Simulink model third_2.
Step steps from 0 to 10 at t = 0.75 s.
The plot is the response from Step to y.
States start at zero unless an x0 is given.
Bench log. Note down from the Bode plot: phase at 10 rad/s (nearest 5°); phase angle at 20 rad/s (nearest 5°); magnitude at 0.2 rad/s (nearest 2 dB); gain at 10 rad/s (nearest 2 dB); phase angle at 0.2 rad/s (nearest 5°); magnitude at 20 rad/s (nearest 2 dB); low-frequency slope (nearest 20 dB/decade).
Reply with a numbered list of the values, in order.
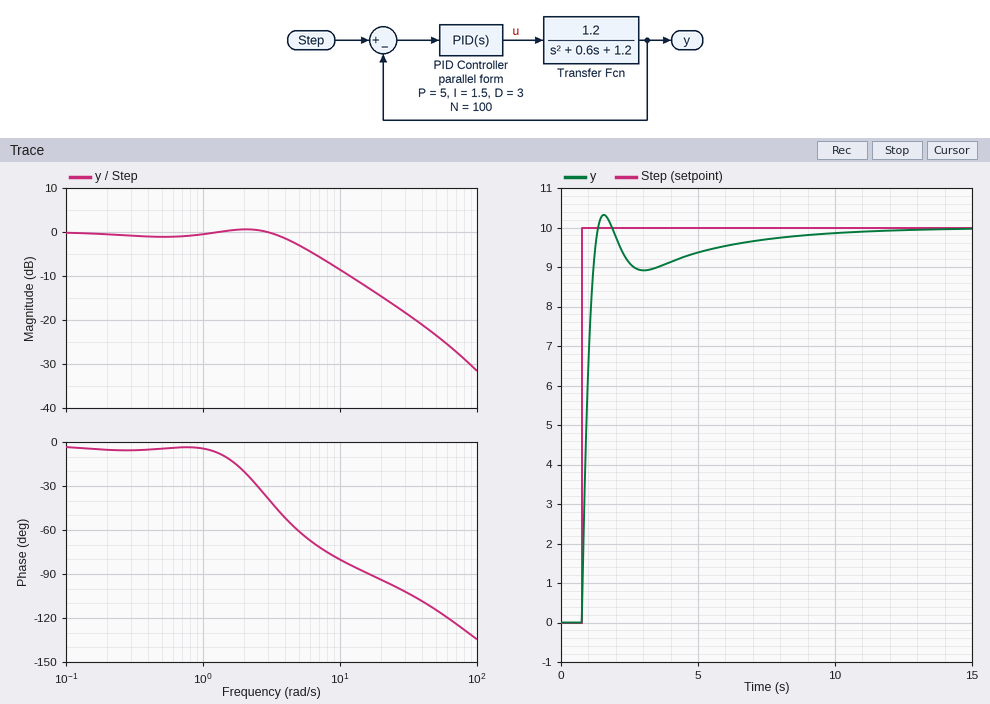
1. -80°
2. -95°
3. 0 dB
4. -8 dB
5. -5°
6. -14 dB
7. 0 dB/decade
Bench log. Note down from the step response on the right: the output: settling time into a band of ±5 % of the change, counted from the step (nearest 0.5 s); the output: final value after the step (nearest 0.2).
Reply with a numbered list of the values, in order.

1. 5.0 s
2. 10.0
